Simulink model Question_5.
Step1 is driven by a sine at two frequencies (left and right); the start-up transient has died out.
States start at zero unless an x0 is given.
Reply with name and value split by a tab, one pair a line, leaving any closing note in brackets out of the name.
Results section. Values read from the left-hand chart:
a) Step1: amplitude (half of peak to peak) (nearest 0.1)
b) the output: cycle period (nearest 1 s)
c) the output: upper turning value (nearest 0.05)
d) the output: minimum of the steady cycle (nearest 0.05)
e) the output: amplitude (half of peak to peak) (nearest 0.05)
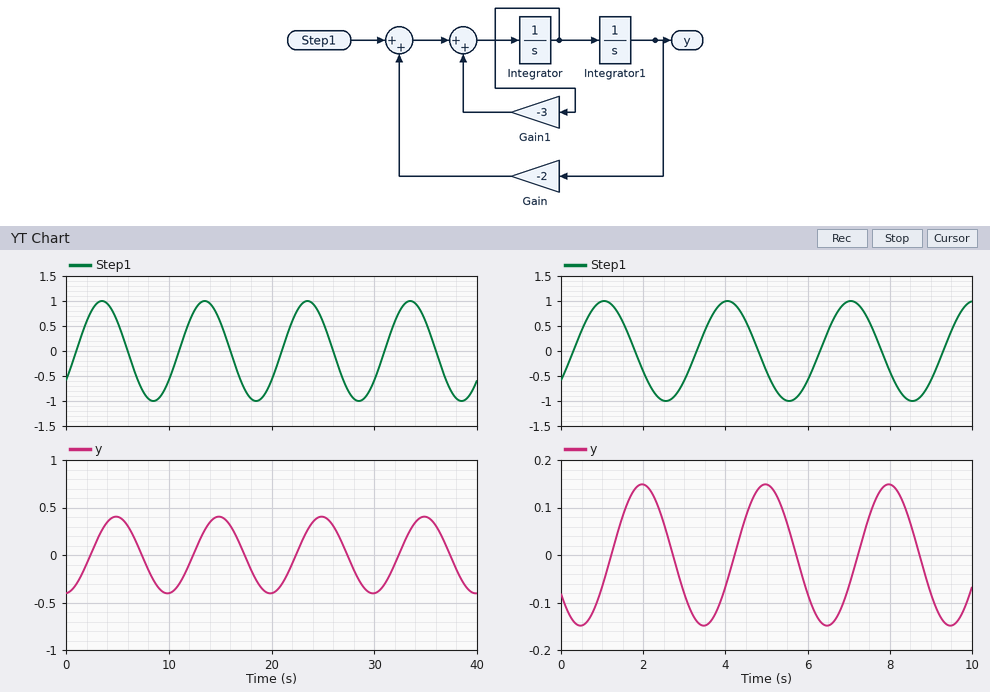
Step1: amplitude (half of peak to peak)	1.0
the output: cycle period	10 s
the output: upper turning value	0.40
the output: minimum of the steady cycle	-0.40
the output: amplitude (half of peak to peak)	0.40
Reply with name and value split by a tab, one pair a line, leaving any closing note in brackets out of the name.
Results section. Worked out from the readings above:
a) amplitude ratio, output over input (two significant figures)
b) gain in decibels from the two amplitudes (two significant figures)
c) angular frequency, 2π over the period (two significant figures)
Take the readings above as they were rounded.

amplitude ratio, output over input	0.40
gain in decibels from the two amplitudes	-8.0 dB
angular frequency, 2π over the period	0.63 rad/s
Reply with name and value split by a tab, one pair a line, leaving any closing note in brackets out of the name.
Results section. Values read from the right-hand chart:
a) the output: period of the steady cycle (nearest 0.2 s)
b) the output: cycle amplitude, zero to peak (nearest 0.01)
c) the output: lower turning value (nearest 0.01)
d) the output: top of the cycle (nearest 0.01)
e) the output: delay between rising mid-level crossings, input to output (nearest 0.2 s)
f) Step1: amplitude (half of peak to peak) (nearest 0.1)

the output: period of the steady cycle	3.0 s
the output: cycle amplitude, zero to peak	0.15
the output: lower turning value	-0.15
the output: top of the cycle	0.15
the output: delay between rising mid-level crossings, input to output	1.0 s
Step1: amplitude (half of peak to peak)	1.0
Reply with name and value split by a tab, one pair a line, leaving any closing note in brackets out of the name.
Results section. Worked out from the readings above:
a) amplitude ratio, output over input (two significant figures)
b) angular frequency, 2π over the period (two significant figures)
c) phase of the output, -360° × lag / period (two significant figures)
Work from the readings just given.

amplitude ratio, output over input	0.15
angular frequency, 2π over the period	2.1 rad/s
phase of the output, -360° × lag / period	-120°
